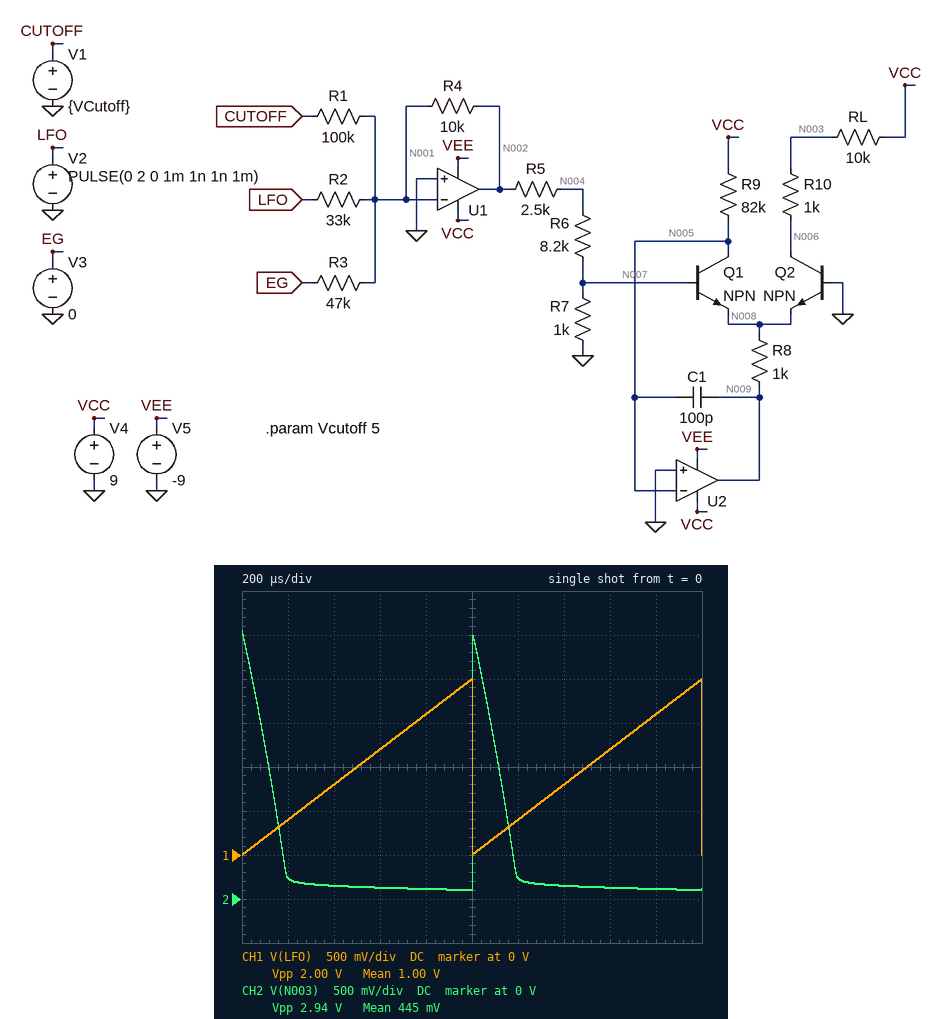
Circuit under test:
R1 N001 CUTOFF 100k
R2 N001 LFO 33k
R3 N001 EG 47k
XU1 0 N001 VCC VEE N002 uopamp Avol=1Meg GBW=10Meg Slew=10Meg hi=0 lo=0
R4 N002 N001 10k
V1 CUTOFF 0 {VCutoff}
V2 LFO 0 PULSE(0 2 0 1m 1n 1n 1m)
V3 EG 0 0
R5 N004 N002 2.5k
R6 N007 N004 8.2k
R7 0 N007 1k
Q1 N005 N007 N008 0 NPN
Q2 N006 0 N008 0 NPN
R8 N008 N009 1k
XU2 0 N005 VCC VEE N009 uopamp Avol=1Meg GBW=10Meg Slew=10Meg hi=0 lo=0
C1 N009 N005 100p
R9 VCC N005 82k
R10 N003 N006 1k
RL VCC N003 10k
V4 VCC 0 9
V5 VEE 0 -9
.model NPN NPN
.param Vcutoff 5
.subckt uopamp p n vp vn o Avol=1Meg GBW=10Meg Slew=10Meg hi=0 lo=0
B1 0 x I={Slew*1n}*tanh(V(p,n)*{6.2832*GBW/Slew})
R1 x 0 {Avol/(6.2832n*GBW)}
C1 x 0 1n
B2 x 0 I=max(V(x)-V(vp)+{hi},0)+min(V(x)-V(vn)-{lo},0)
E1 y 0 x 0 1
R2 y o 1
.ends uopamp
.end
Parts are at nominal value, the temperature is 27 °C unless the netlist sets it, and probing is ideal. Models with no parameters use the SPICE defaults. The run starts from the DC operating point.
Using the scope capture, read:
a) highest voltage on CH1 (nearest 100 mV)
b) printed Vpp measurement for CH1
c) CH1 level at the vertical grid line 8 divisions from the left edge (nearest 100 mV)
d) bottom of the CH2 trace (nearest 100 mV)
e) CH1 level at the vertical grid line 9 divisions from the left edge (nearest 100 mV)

2.0 V
2.00 V
1.2 V
100 mV
1.6 V
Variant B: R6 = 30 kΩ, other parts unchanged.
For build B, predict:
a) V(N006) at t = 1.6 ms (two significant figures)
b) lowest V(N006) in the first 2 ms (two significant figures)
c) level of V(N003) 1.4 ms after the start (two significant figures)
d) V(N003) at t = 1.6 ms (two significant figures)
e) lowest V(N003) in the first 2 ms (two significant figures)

5.6 V
4.5 V
6.3 V
5.9 V
4.9 V
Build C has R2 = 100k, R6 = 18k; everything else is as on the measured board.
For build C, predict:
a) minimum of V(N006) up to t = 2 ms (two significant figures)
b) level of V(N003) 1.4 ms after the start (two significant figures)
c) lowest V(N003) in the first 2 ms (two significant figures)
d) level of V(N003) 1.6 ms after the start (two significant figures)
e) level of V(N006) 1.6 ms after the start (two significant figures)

4.6 V
5.8 V
5.0 V
5.5 V
5.2 V
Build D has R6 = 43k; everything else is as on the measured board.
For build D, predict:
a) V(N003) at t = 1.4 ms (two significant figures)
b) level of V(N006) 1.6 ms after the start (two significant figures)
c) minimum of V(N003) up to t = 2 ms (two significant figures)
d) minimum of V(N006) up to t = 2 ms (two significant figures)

6.9 V
6.4 V
6.1 V
5.8 V
